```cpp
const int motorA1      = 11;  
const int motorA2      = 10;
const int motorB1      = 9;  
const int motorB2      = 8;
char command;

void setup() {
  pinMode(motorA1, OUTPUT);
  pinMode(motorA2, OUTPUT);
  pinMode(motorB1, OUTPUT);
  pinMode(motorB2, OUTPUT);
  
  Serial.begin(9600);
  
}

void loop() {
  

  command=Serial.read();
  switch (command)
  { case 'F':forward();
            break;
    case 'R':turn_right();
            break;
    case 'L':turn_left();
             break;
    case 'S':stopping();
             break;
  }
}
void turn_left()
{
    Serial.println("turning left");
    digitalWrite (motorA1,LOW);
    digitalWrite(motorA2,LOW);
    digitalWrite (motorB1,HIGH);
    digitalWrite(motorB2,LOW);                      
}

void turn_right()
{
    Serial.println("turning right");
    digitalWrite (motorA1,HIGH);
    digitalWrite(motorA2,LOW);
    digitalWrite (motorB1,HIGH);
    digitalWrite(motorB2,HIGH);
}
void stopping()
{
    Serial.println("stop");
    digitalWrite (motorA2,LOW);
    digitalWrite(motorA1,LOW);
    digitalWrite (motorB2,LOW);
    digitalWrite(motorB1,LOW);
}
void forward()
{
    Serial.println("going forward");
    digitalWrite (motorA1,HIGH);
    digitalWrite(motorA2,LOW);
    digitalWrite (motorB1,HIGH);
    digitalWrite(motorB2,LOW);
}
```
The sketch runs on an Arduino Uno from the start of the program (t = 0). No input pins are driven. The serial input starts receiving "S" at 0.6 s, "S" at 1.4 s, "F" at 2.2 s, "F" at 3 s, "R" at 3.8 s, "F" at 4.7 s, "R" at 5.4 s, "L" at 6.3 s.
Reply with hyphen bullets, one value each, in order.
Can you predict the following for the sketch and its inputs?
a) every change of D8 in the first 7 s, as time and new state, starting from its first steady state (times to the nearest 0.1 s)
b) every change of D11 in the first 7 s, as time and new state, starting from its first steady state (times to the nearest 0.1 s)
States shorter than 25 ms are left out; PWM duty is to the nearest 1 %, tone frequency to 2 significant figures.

- 0 s low; 3.8 s high; 4.7 s low; 5.4 s high; 6.3 s low
- 0 s low; 2.2 s high; 6.3 s low
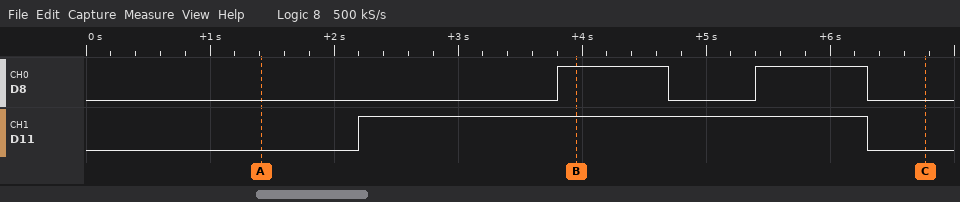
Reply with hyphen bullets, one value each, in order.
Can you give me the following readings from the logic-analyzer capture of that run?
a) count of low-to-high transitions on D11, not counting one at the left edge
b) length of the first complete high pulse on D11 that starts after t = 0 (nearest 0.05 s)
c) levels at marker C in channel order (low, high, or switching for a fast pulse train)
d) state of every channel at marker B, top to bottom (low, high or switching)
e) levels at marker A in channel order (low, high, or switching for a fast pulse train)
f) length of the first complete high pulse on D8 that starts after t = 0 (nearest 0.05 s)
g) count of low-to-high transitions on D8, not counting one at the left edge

- 1
- 4.10 s
- D8 low, D11 low
- D8 high, D11 high
- D8 low, D11 low
- 0.90 s
- 2
